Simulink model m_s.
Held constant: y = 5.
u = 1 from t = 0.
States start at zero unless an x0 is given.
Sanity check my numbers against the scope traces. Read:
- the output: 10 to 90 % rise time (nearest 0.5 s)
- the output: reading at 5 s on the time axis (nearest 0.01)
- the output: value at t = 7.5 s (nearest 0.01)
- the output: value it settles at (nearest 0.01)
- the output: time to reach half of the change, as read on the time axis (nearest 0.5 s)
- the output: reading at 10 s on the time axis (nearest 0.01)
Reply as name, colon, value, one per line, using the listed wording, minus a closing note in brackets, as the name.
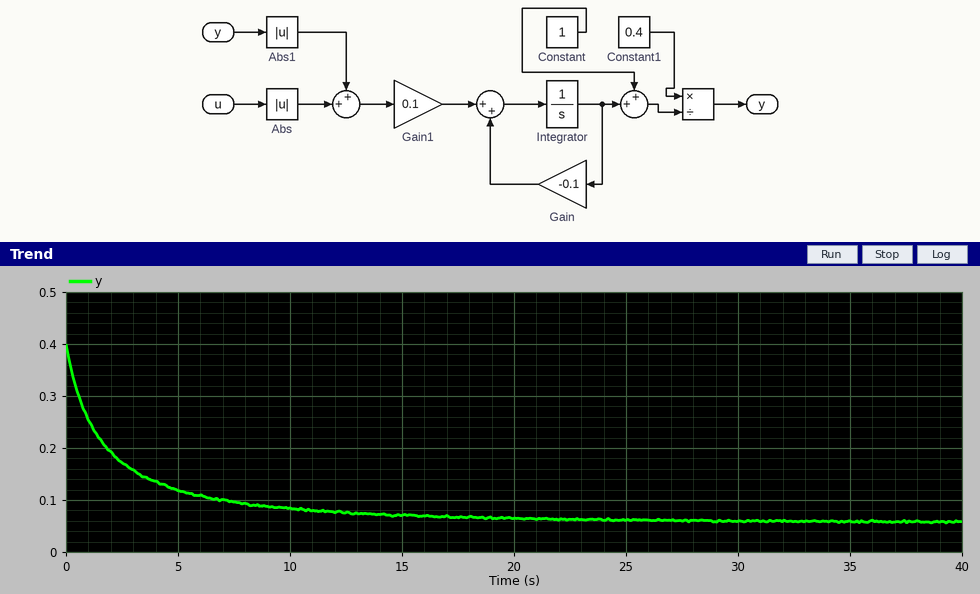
the output: 10 to 90 % rise time: 8.0 s
the output: reading at 5 s on the time axis: 0.12
the output: value at t = 7.5 s: 0.10
the output: value it settles at: 0.06
the output: time to reach half of the change, as read on the time axis: 1.5 s
the output: reading at 10 s on the time axis: 0.08
